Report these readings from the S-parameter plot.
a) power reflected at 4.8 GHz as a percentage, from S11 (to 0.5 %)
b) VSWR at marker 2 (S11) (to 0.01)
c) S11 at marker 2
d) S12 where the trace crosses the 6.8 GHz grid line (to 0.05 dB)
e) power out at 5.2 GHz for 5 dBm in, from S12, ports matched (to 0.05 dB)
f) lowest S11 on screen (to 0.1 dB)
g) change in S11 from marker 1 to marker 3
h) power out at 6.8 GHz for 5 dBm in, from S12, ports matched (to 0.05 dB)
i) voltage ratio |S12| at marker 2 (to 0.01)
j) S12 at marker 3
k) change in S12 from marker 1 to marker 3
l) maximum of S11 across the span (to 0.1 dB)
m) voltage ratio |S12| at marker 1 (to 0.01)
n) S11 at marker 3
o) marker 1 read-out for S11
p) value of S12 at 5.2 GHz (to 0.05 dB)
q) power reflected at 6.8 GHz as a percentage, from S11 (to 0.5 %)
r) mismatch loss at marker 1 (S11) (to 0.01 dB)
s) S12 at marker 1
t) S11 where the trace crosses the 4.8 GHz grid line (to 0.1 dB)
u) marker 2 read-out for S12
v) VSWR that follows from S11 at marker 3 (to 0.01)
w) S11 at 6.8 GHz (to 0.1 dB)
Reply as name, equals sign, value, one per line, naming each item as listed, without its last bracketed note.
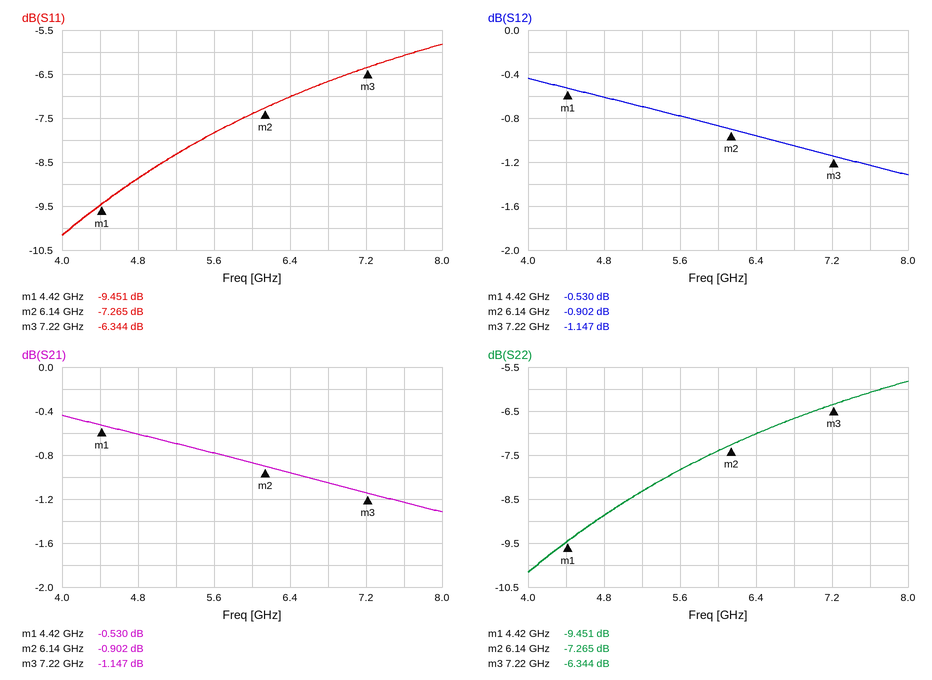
power reflected at 4.8 GHz as a percentage, from S11 = 13.0 %
VSWR at marker 2 (S11) = 2.53
S11 at marker 2 = -7.265 dB
S12 where the trace crosses the 6.8 GHz grid line = -1.05 dB
power out at 5.2 GHz for 5 dBm in, from S12, ports matched = 4.30 dBm
lowest S11 on screen = -10.2 dB
change in S11 from marker 1 to marker 3 = 3.107 dB
power out at 6.8 GHz for 5 dBm in, from S12, ports matched = 3.95 dBm
voltage ratio |S12| at marker 2 = 0.90
S12 at marker 3 = -1.147 dB
change in S12 from marker 1 to marker 3 = -0.617 dB
maximum of S11 across the span = -5.8 dB
voltage ratio |S12| at marker 1 = 0.94
S11 at marker 3 = -6.344 dB
marker 1 read-out for S11 = -9.451 dB
value of S12 at 5.2 GHz = -0.70 dB
power reflected at 6.8 GHz as a percentage, from S11 = 21.5 %
mismatch loss at marker 1 (S11) = 0.52 dB
S12 at marker 1 = -0.530 dB
S11 where the trace crosses the 4.8 GHz grid line = -8.9 dB
marker 2 read-out for S12 = -0.902 dB
VSWR that follows from S11 at marker 3 = 2.86
S11 at 6.8 GHz = -6.7 dB
